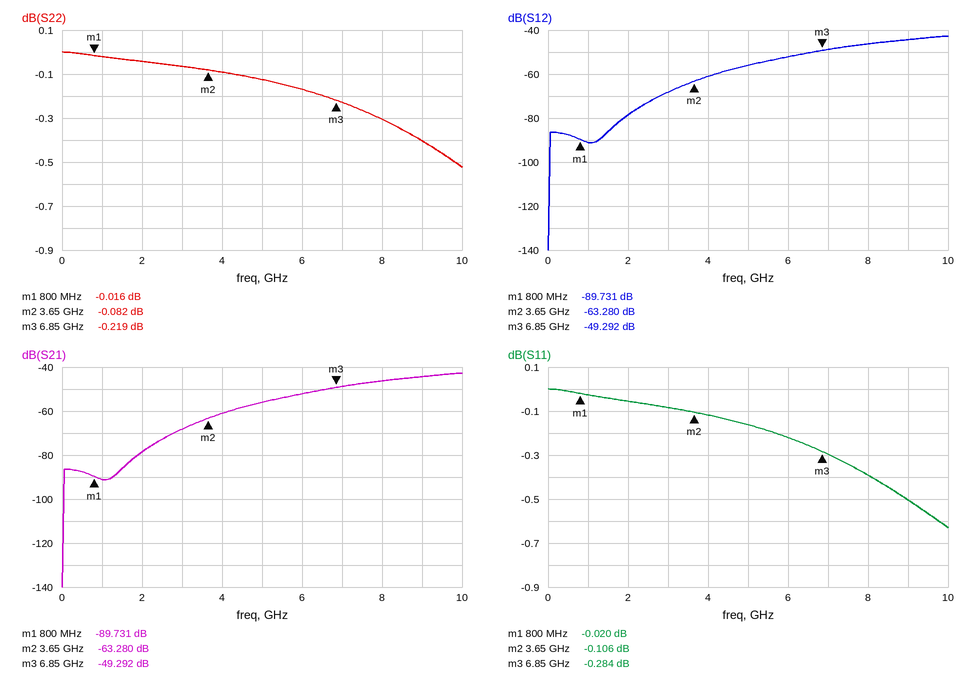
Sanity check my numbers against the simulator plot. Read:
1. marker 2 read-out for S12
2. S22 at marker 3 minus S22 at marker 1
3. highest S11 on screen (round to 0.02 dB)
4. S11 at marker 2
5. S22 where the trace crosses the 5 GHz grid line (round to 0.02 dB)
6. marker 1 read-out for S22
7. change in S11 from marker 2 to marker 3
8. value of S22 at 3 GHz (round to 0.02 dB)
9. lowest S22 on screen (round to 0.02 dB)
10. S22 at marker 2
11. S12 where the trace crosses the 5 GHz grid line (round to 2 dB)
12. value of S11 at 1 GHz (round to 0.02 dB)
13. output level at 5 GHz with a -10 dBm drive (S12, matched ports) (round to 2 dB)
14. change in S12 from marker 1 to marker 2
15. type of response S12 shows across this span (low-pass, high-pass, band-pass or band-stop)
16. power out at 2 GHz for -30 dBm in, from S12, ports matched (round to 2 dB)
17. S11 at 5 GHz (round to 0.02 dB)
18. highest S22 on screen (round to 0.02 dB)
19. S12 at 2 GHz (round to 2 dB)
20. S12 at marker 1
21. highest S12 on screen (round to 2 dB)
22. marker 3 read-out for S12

-63.280 dB
-0.203 dB
0.00 dB
-0.106 dB
-0.12 dB
-0.016 dB
-0.178 dB
-0.06 dB
-0.52 dB
-0.082 dB
-56 dB
-0.02 dB
-66 dBm
26.451 dB
high-pass
-108 dBm
-0.16 dB
0.00 dB
-78 dB
-89.731 dB
-42 dB
-49.292 dB
